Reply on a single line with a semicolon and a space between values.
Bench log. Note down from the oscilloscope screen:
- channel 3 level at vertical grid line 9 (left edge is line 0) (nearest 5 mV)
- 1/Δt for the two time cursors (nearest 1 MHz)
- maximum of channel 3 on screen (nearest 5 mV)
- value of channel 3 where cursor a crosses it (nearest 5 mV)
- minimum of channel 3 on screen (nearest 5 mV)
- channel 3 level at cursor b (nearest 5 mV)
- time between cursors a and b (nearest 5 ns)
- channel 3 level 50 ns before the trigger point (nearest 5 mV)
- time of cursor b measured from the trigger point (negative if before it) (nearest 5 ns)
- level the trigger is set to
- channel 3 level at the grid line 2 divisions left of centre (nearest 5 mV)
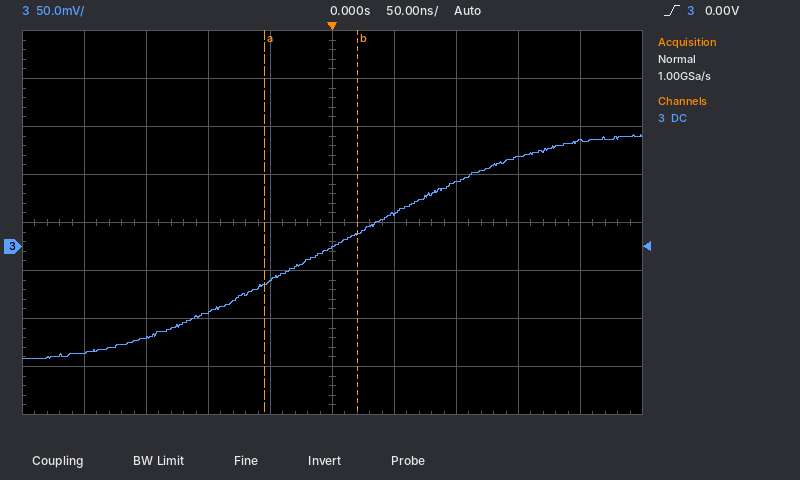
110 mV; 13 MHz; 115 mV; -40 mV; -115 mV; 15 mV; 75 ns; -35 mV; +20 ns; 0.00 V; -70 mV
